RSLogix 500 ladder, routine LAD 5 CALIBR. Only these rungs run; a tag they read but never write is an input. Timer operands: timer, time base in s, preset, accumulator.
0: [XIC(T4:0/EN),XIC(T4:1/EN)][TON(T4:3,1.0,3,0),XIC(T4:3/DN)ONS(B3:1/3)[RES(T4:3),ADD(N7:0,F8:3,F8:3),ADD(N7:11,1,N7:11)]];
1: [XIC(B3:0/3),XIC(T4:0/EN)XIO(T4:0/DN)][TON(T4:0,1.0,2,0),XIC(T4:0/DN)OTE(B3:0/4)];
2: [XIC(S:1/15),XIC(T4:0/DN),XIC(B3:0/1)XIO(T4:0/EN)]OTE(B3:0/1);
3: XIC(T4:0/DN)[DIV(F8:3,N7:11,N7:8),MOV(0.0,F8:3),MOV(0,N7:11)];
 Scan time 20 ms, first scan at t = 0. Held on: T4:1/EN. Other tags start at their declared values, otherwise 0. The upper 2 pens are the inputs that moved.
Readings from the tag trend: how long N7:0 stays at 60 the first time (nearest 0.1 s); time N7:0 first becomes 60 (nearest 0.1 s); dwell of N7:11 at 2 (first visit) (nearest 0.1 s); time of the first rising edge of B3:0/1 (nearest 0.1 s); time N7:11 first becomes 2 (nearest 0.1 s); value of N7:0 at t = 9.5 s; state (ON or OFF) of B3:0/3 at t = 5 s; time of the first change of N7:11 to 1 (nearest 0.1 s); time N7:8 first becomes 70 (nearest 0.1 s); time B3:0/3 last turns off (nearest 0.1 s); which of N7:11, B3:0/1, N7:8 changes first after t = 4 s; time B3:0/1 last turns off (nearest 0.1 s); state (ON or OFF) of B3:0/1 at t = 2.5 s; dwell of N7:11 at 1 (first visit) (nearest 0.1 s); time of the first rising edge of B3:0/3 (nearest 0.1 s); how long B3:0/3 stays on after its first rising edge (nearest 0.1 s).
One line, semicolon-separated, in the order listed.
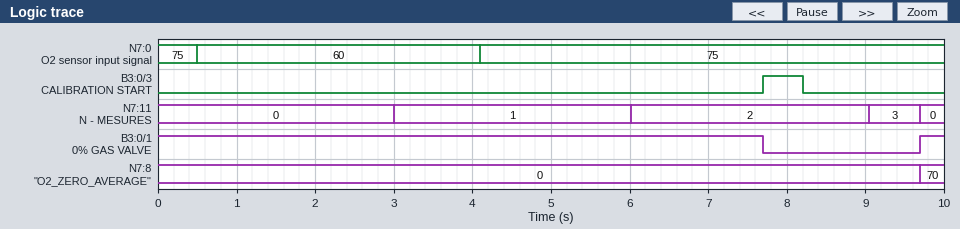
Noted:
3.6 s; 0.5 s; 3.0 s; 9.7 s; 6.0 s; 75; OFF; 3.0 s; 9.7 s; 8.2 s; N7:11; 7.7 s; ON; 3.0 s; 7.7 s; 0.5 s
